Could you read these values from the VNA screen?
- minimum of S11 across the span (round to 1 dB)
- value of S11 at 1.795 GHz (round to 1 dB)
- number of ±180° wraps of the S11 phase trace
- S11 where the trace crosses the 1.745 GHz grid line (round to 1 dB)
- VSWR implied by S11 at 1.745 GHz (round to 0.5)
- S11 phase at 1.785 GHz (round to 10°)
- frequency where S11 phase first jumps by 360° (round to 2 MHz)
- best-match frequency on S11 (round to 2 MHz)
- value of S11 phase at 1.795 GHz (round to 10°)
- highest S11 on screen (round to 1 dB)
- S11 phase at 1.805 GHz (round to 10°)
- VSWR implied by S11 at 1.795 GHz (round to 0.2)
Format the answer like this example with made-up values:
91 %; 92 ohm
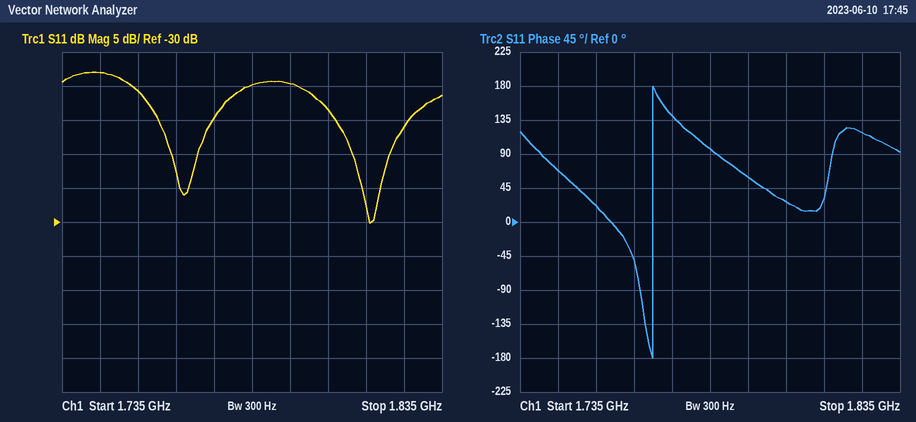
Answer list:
-30 dB; -10 dB; 1; -8 dB; 2.5; 100°; 1.770 GHz; 1.816 GHz; 60°; -8 dB; 30°; 2.0
